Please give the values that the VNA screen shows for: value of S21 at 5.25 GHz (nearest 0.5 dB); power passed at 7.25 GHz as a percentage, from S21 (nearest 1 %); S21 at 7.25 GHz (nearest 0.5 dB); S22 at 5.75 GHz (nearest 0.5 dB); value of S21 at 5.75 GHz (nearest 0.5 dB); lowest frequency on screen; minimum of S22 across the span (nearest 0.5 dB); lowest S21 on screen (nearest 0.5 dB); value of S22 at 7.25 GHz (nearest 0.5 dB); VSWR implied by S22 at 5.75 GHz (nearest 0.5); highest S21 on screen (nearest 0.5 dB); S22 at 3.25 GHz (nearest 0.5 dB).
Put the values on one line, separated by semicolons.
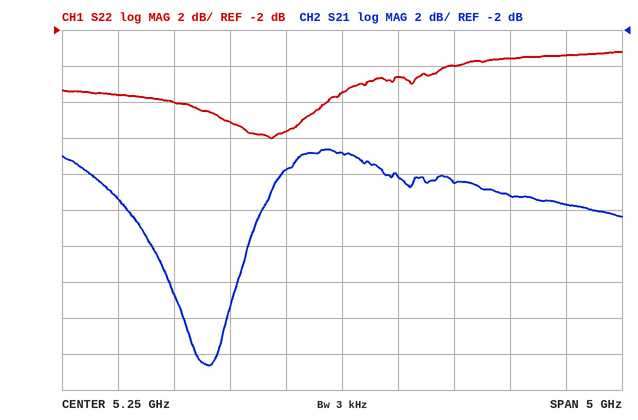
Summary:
-9.0 dB; 7 %; -11.5 dB; -4.5 dB; -10.0 dB; 2.75 GHz; -8.0 dB; -20.5 dB; -3.5 dB; 4.0; -8.5 dB; -5.5 dB
